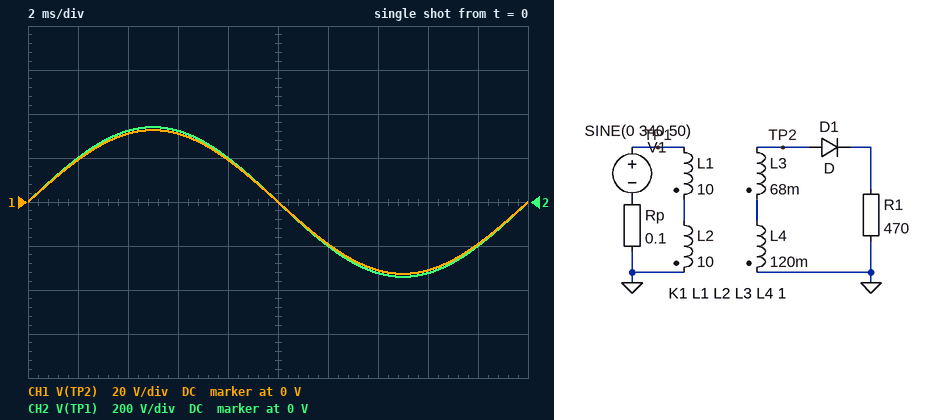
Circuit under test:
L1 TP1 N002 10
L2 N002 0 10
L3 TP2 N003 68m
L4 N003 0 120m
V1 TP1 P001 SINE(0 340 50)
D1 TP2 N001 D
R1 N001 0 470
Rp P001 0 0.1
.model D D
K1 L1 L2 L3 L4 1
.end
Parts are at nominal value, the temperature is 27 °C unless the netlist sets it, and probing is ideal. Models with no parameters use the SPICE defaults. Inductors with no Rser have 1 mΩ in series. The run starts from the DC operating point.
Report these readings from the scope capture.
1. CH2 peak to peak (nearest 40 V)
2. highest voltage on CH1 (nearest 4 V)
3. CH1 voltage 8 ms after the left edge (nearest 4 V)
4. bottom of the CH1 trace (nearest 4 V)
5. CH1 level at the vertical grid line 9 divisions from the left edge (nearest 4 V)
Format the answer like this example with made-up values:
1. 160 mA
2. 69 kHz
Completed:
1. 680 V
2. 32 V
3. 20 V
4. -32 V
5. -20 V
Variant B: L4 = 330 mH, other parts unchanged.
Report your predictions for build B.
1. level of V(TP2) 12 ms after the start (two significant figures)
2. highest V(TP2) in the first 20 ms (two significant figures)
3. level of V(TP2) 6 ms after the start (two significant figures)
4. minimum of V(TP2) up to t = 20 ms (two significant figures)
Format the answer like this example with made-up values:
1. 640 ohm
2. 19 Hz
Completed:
1. -26 V
2. 45 V
3. 43 V
4. -45 V
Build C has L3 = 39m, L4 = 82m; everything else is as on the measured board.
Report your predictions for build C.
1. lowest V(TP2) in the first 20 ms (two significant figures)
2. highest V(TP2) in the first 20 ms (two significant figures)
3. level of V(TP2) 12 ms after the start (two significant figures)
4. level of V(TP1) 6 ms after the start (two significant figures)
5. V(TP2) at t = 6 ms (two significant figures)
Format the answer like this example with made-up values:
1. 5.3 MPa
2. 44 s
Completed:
1. -26 V
2. 26 V
3. -15 V
4. 320 V
5. 25 V
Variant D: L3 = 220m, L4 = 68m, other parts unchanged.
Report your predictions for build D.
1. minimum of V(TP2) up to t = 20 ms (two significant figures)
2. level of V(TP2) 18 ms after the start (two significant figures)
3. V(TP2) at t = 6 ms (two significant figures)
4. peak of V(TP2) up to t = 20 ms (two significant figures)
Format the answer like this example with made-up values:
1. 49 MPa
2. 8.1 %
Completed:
1. -39 V
2. -23 V
3. 37 V
4. 39 V
